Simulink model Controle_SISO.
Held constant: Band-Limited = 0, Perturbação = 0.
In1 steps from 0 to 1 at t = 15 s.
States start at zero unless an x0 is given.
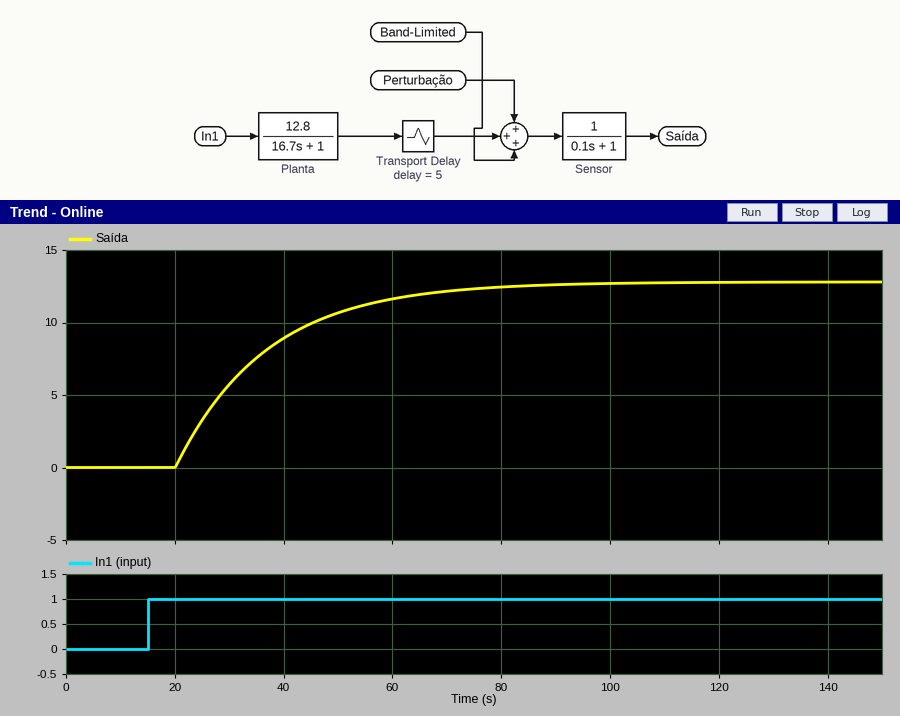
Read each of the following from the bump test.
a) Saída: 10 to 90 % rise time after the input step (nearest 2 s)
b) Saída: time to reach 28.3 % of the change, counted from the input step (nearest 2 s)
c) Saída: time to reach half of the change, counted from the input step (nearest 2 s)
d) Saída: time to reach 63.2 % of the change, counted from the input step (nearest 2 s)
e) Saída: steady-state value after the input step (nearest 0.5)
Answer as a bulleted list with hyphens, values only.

- 36 s
- 10 s
- 16 s
- 22 s
- 13.0
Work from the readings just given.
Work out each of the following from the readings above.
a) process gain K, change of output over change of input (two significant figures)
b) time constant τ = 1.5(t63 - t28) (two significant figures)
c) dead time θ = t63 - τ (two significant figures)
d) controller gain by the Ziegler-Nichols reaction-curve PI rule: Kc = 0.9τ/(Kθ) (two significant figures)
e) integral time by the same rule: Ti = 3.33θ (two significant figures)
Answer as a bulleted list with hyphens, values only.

- 13
- 18 s
- 4.0 s
- 0.31
- 13 s
